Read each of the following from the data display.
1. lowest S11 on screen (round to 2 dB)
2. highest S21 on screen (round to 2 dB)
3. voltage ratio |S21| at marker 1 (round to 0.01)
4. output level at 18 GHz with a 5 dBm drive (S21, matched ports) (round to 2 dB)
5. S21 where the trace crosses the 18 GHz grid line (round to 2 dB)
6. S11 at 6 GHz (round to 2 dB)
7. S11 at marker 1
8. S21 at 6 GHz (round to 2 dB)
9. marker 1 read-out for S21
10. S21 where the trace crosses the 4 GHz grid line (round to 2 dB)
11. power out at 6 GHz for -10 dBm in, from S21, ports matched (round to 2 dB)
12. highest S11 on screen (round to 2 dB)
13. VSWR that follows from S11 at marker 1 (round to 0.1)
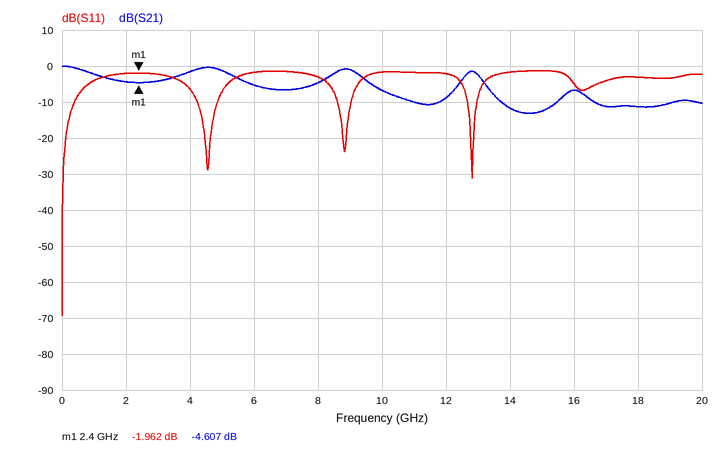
-70 dB
0 dB
0.59
-6 dBm
-12 dB
-2 dB
-1.962 dB
-6 dB
-4.607 dB
-2 dB
-16 dBm
-2 dB
8.9
